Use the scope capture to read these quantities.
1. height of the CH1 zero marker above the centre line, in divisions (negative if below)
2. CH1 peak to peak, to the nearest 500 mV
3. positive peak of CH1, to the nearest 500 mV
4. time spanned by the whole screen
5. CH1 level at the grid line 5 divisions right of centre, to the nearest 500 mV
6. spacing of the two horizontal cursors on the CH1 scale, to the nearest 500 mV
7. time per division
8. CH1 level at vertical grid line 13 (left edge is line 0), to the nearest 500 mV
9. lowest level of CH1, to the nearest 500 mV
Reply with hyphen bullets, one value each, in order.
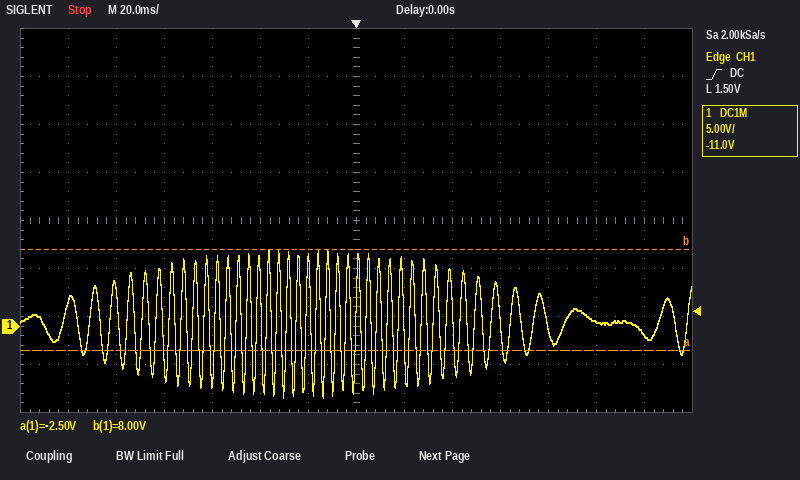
- -2.2 div
- 15.5 V
- 8.0 V
- 280 ms
- 500 mV
- 10.5 V
- 20 ms
- -1.0 V
- -7.5 V
